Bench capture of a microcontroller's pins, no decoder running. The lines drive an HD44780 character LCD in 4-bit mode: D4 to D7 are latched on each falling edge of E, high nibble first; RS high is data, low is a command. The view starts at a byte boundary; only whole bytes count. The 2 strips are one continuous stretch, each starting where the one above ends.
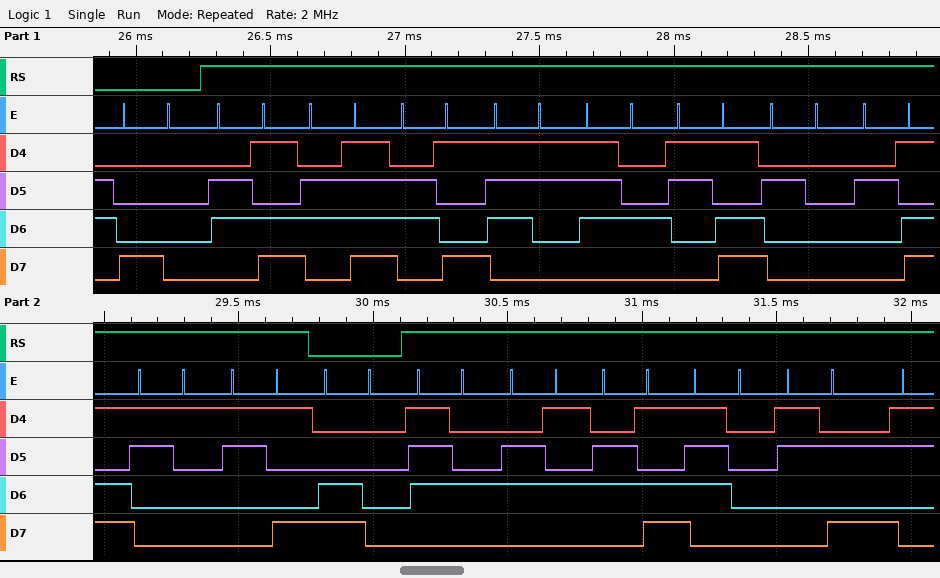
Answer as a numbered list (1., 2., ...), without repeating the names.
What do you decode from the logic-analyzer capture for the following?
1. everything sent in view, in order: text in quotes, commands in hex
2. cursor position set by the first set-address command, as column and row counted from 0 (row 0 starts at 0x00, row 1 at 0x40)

1. 0x80 "moist= -19" 0xC0 "temp:"
2. column 0, row 0
